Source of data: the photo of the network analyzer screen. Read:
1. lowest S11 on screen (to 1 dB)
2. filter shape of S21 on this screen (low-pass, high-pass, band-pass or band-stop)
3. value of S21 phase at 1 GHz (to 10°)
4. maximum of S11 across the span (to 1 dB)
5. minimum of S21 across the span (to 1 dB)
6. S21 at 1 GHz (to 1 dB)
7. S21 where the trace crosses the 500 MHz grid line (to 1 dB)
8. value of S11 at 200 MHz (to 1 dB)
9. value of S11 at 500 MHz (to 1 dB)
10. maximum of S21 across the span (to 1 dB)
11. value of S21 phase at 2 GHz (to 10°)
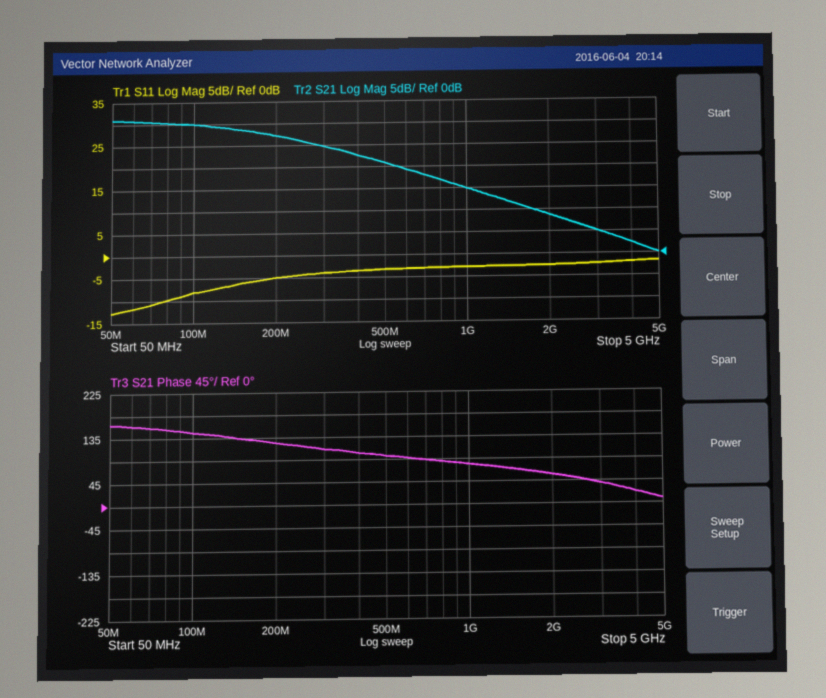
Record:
-13 dB
low-pass
80°
-2 dB
0 dB
15 dB
21 dB
-5 dB
-3 dB
31 dB
60°
